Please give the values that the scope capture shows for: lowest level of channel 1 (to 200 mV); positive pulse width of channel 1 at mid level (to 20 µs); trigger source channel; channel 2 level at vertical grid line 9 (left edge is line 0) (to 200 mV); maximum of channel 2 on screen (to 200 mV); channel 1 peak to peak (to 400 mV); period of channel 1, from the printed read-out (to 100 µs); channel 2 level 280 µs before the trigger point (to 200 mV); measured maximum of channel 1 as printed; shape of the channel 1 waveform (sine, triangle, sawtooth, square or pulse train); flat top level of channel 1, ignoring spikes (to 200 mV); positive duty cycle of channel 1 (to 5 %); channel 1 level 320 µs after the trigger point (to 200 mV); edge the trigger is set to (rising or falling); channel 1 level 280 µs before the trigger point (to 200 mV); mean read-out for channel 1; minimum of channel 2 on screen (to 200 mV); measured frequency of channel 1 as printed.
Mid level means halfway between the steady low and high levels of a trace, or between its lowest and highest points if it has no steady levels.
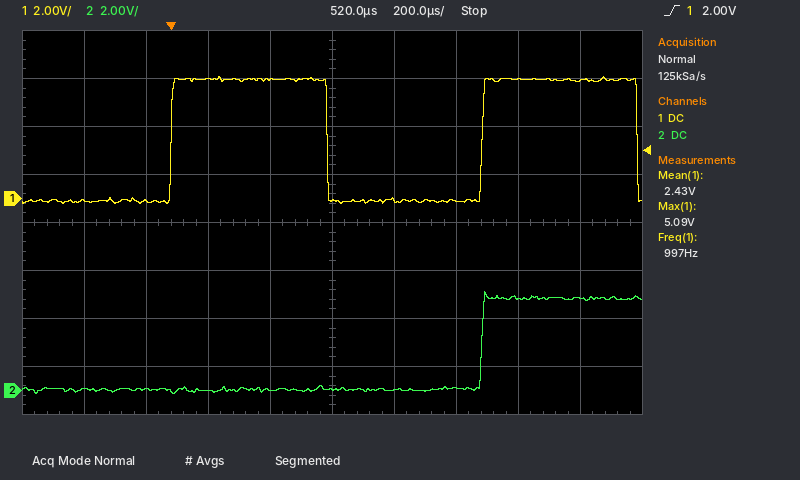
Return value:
-200 mV
500 µs
channel 1
3.8 V
4.2 V
5.2 V
1.0 ms
0.0 V
5.09 V
square
5.0 V
50 %
5.0 V
rising
0.0 V
2.43 V
-200 mV
997 Hz
